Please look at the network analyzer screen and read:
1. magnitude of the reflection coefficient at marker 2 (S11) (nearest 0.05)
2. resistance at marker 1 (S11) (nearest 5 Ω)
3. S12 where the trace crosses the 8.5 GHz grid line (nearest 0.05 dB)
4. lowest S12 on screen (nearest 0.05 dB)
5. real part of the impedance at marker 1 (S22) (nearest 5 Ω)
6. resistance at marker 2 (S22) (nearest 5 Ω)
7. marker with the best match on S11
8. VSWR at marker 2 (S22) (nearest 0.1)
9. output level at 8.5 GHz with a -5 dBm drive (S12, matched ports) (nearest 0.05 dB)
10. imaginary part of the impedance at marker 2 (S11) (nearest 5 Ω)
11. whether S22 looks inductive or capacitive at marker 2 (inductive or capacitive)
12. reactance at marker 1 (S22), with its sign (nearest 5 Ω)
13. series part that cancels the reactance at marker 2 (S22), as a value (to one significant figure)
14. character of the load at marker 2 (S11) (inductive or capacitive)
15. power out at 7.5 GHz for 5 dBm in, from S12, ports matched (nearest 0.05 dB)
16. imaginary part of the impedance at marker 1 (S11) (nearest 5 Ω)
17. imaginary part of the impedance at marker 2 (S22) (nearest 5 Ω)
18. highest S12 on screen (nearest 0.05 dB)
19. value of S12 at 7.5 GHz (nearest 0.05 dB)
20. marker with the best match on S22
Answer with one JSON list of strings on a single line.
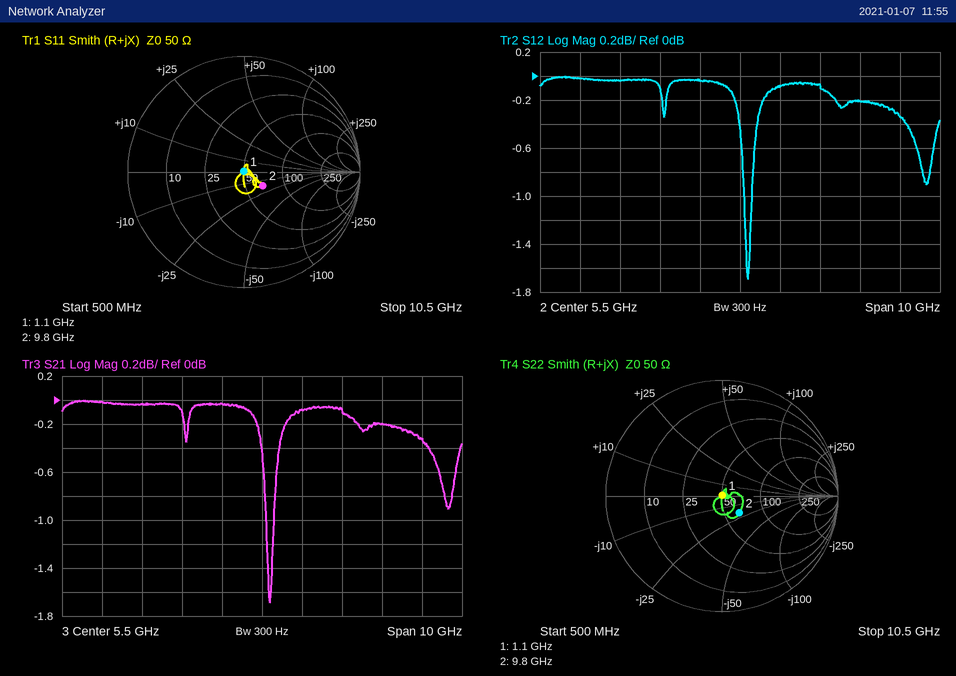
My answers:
["0.20", "50 Ω", "-0.20 dB", "-1.70 dB", "50 Ω", "65 Ω", "marker 1", "1.5", "-5.20 dBm", "-15 Ω", "capacitive", "0 Ω", "300 pH", "capacitive", "4.90 dBm", "0 Ω", "-20 Ω", "0.00 dB", "-0.10 dB", "marker 1"]
